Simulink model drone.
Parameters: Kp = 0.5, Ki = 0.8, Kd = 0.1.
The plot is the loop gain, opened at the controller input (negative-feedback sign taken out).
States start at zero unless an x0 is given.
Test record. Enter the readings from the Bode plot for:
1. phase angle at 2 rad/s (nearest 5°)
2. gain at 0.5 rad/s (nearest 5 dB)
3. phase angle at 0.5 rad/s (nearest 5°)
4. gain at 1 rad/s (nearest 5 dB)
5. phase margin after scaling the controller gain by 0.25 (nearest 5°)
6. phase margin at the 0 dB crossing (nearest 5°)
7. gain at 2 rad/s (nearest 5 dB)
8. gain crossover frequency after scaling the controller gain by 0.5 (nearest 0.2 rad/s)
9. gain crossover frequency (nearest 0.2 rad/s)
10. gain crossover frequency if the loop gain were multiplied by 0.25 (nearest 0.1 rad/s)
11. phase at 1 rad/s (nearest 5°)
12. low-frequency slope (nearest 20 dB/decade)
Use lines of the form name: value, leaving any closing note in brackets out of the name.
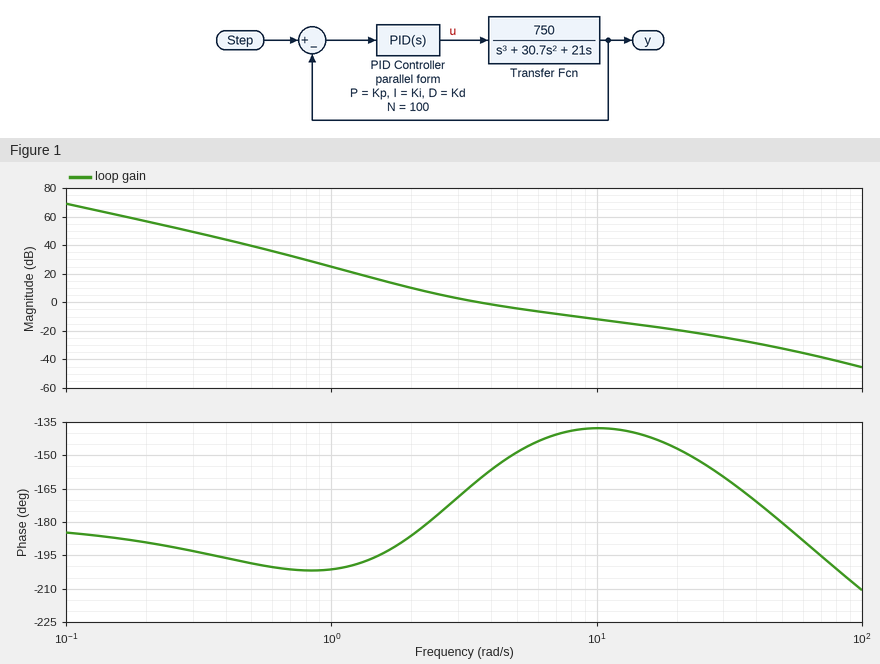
phase angle at 2 rad/s: -185°
gain at 0.5 rad/s: 40 dB
phase angle at 0.5 rad/s: -200°
gain at 1 rad/s: 25 dB
phase margin after scaling the controller gain by 0.25: -10°
phase margin at the 0 dB crossing: 20°
gain at 2 rad/s: 10 dB
gain crossover frequency after scaling the controller gain by 0.5: 2.4 rad/s
gain crossover frequency: 3.6 rad/s
gain crossover frequency if the loop gain were multiplied by 0.25: 1.8 rad/s
phase at 1 rad/s: -200°
low-frequency slope: -40 dB/decade
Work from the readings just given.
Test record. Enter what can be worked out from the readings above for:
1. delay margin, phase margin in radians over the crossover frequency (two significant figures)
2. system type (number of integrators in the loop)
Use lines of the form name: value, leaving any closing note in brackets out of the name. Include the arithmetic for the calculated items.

delay margin, phase margin in radians over the crossover frequency: 20 × π / 180 / 3.6 = 0.097 s
system type: 2
